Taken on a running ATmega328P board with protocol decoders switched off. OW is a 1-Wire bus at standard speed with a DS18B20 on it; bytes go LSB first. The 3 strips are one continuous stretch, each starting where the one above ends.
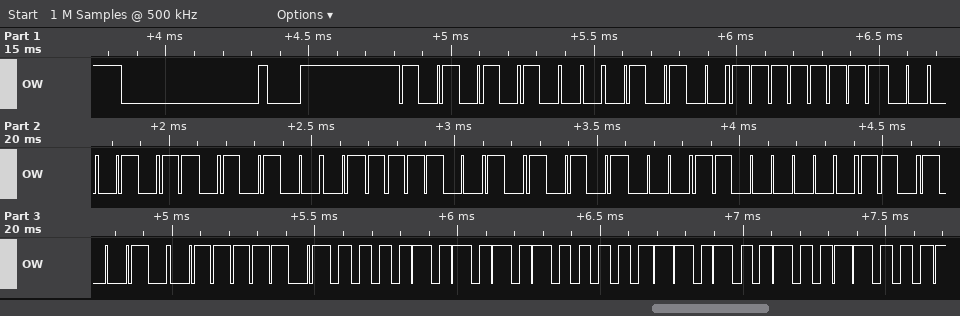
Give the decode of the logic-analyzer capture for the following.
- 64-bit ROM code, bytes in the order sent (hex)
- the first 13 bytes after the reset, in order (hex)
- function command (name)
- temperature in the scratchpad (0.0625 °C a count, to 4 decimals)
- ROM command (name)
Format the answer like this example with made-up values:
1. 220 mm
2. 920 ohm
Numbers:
1. 28 FF D0 8A 4F 15 03 4B
2. 55 28 FF D0 8A 4F 15 03 4B BE 50 05 4B
3. Read Scratchpad
4. 85.0000 °C
5. Match ROM
